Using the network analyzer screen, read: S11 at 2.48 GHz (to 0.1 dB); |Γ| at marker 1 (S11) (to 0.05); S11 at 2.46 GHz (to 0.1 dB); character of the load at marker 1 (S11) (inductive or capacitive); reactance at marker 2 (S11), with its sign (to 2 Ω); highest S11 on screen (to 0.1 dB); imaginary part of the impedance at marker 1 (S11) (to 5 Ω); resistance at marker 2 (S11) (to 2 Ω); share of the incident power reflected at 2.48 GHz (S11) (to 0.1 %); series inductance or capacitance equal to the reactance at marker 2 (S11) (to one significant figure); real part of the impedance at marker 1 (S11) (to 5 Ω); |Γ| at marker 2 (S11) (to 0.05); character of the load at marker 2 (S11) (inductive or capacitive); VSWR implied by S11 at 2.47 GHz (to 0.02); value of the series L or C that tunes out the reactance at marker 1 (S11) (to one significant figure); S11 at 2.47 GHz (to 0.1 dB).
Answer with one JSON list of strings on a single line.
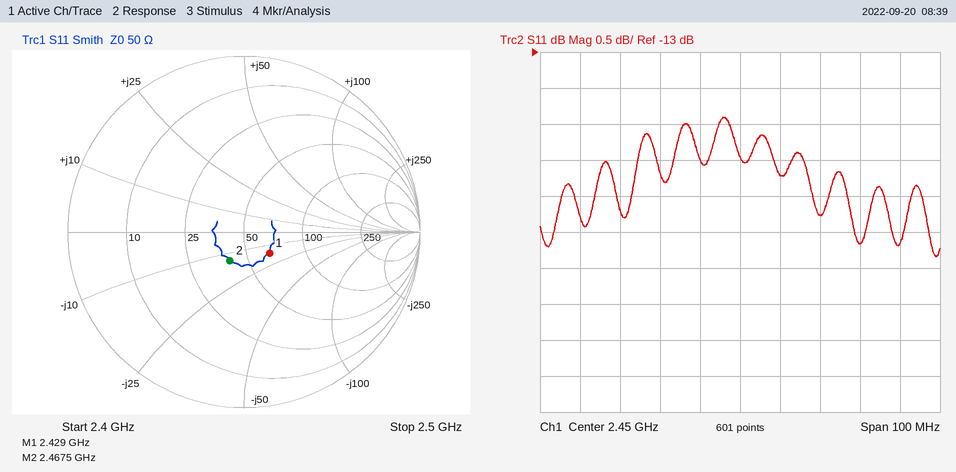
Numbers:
["-15.7 dB", "0.20", "-14.7 dB", "capacitive", "-14 Ω", "-13.9 dB", "-15 Ω", "40 Ω", "2.7 %", "5 pF", "65 Ω", "0.20", "capacitive", "1.42", "1 nH", "-15.3 dB"]
